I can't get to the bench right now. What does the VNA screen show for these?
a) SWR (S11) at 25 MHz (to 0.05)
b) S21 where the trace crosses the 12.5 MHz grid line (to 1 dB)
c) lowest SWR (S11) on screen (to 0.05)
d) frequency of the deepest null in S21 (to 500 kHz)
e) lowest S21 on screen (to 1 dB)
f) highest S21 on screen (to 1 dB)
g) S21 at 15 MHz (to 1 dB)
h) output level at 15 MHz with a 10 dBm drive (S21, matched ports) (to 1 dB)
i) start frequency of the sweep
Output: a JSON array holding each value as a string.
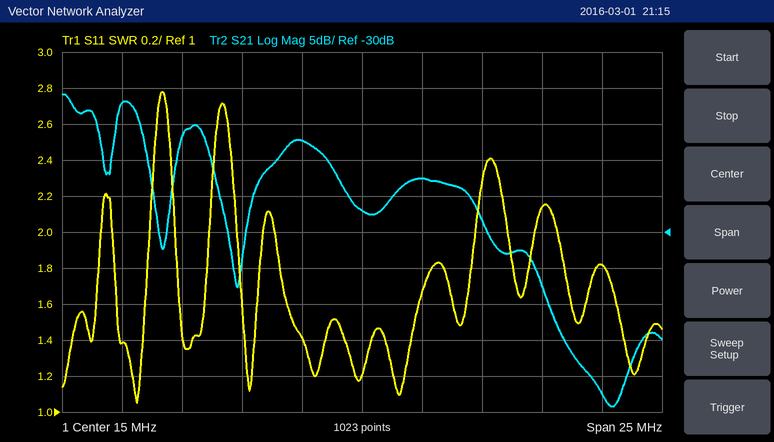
["1.80", "-17 dB", "1.05", "25.5 MHz", "-54 dB", "-11 dB", "-27 dB", "-17 dBm", "2.5 MHz"]
